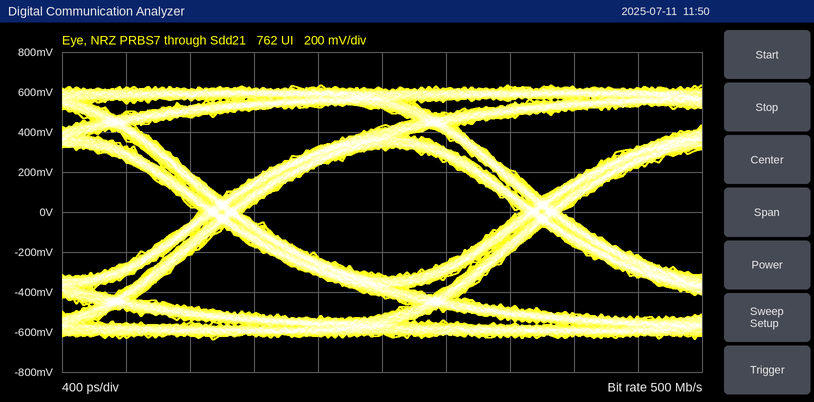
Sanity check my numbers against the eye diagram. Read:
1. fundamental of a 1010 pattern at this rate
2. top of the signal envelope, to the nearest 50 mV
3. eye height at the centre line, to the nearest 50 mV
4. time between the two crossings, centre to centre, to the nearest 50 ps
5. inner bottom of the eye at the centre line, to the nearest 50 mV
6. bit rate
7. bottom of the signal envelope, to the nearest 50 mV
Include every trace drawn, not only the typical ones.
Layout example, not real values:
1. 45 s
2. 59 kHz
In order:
1. 250 MHz
2. 650 mV
3. 650 mV
4. 2.00 ns
5. -300 mV
6. 500 Mb/s
7. -650 mV
